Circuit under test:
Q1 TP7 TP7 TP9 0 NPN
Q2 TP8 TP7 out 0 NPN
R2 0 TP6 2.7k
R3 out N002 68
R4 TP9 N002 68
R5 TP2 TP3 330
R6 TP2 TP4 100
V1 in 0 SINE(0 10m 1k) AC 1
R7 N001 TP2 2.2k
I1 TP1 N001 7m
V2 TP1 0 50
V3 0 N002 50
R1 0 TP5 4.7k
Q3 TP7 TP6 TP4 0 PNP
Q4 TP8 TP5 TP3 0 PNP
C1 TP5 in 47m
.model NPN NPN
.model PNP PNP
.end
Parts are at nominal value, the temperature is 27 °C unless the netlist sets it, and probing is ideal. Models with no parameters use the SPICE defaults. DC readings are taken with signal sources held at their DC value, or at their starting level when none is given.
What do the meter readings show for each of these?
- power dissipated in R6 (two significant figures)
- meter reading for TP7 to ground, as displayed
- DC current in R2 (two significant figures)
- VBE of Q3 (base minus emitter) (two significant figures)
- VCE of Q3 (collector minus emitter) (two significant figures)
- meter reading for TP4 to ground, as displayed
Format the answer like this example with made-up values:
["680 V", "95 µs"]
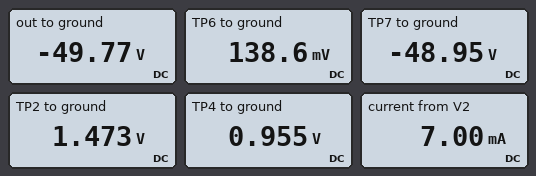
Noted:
["2.7 mW", "-48.95 V", "51 µA", "-820 mV", "-50 V", "0.955 V"]
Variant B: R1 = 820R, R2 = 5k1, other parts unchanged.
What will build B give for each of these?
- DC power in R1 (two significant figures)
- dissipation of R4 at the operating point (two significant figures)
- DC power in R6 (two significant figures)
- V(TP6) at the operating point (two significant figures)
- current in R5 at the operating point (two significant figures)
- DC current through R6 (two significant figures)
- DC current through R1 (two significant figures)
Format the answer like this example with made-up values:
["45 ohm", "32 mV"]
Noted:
["390 nW", "840 µW", "2.3 mW", "240 mV", "2.2 mA", "4.8 mA", "22 µA"]
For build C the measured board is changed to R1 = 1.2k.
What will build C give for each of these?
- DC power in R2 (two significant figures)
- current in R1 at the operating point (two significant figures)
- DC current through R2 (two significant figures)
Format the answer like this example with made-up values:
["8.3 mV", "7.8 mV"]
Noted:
["6.8 µW", "19 µA", "50 µA"]
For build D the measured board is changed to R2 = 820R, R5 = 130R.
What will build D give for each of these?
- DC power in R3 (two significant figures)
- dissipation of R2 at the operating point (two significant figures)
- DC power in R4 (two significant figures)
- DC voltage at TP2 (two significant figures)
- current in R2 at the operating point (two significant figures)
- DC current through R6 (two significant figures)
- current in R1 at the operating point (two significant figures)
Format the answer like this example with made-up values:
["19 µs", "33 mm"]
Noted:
["800 µW", "1.5 µW", "830 µW", "1.3 V", "43 µA", "4.3 mA", "27 µA"]
